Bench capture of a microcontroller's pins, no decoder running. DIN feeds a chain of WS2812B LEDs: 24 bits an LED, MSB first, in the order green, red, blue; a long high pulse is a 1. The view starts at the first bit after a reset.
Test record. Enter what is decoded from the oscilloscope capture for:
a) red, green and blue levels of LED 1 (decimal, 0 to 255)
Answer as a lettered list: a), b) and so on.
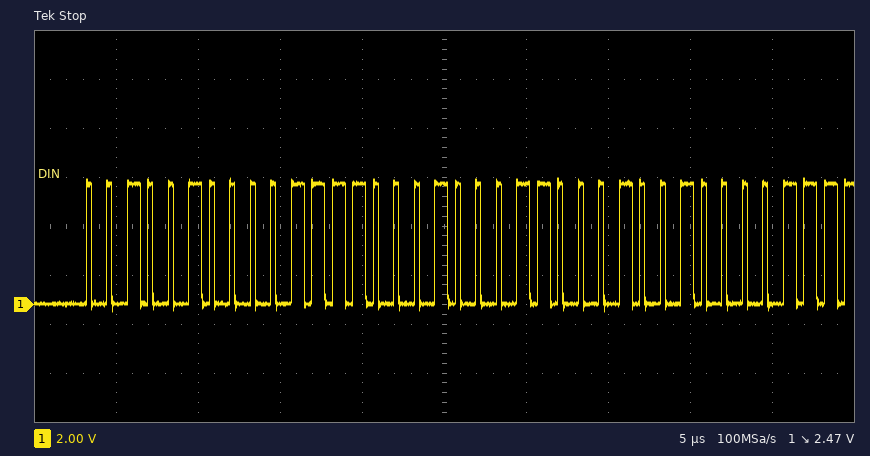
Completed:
a) 60, 36, 70
